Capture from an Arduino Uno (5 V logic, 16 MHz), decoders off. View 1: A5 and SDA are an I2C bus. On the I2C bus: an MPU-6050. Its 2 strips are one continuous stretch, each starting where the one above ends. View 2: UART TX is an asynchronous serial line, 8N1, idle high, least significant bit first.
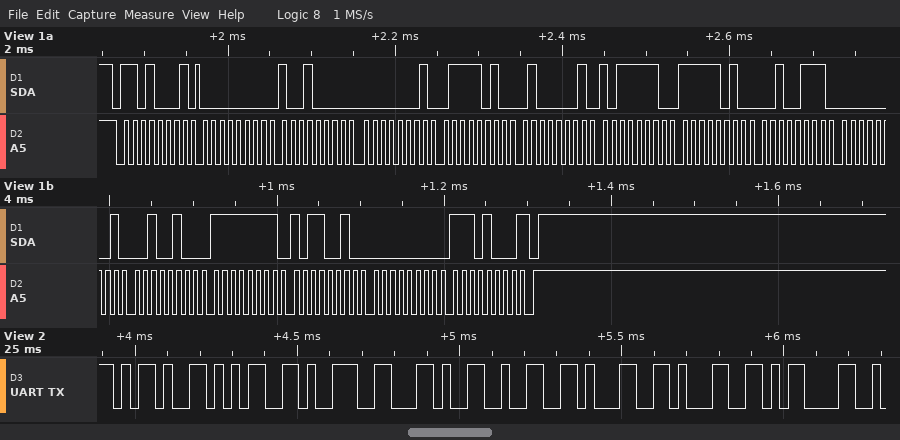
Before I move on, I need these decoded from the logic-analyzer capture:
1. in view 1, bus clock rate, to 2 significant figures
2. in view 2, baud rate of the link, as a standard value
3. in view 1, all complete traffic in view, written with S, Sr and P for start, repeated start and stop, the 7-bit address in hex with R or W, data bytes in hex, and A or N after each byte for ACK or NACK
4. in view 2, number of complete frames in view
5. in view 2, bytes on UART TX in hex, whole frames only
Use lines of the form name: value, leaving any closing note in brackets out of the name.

in view 1, bus clock rate, to 2 significant figures: 100 kHz
in view 2, baud rate of the link, as a standard value: 38400 baud
in view 1, all complete traffic in view, written with S, Sr and P for start, repeated start and stop, the 7-bit address in hex with R or W, data bytes in hex, and A or N after each byte for ACK or NACK: S 68R A 00 A 90 A 01 A 7A A 41 A BE A FA A 27 A 01 A 24 A FF A B2 A 00 A E8 N P
in view 2, number of complete frames in view: 8
in view 2, bytes on UART TX in hex, whole frames only: 0x2D 0x35 0x39 0x2C 0x32 0x31 0x31 0x0D
